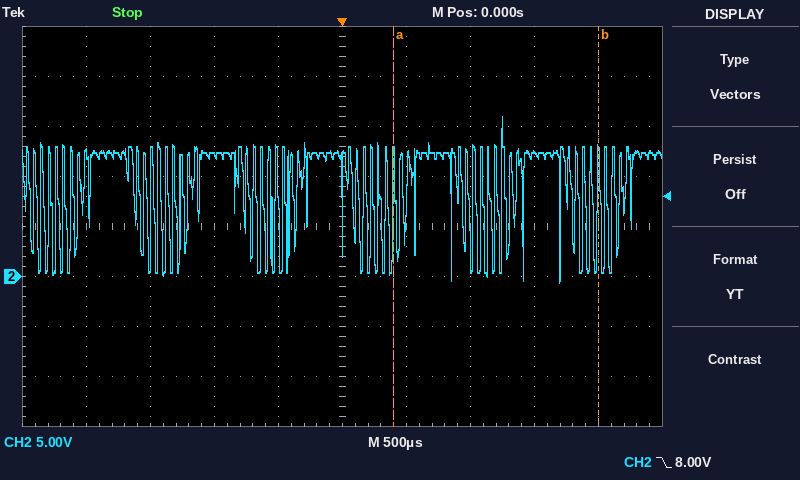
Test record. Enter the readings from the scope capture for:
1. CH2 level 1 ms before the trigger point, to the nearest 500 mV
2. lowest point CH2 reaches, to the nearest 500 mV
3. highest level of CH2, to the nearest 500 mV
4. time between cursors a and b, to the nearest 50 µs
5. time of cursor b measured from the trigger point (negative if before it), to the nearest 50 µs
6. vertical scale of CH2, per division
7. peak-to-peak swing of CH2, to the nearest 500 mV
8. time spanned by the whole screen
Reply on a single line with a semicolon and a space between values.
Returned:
12.0 V; -500 mV; 16.0 V; 1.60 ms; +2.00 ms; 5 V; 16.5 V; 5 ms
